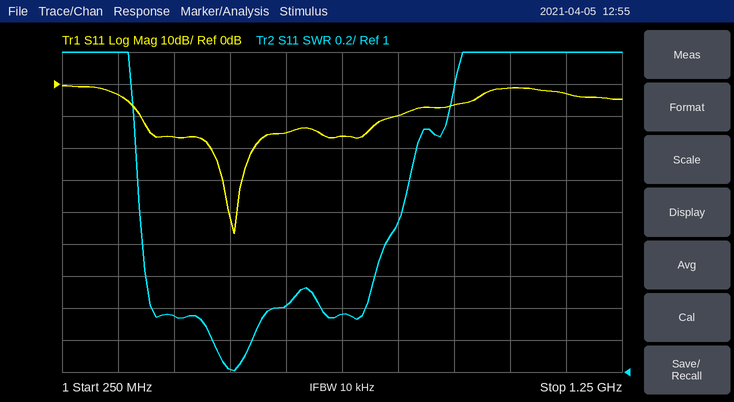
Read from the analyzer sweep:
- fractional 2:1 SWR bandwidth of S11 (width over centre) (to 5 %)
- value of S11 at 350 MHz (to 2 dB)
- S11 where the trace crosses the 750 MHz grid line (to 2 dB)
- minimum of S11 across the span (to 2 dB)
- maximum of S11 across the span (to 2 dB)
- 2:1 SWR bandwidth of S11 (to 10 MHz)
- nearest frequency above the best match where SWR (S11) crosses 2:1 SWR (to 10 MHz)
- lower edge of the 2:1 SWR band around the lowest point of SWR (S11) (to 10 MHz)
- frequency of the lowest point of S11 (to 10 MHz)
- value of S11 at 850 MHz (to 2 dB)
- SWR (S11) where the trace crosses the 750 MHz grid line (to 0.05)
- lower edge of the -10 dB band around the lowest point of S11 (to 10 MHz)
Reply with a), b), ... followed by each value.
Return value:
a) 75 %
b) -4 dB
c) -16 dB
d) -46 dB
e) 0 dB
f) 470 MHz
g) 860 MHz
h) 390 MHz
i) 560 MHz
j) -10 dB
k) 1.35
l) 390 MHz
